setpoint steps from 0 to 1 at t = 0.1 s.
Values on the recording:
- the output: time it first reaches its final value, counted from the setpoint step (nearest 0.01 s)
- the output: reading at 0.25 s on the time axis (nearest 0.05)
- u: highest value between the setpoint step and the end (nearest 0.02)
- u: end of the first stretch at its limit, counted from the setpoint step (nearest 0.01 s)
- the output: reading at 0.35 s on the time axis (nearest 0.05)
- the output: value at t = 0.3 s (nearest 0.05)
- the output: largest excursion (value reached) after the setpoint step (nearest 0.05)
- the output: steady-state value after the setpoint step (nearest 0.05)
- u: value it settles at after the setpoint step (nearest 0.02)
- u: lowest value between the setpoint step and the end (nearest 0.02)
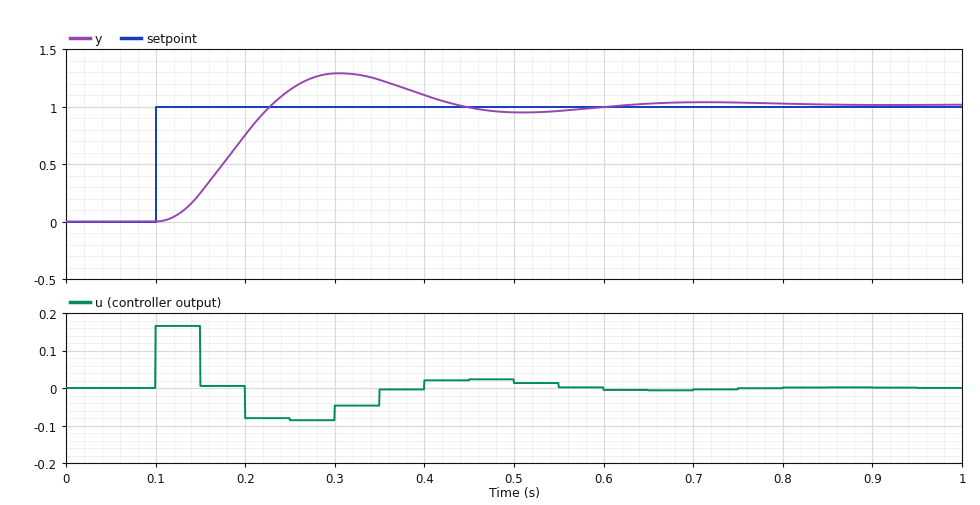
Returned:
0.13 s
1.15
0.16
0.05 s
1.25
1.30
1.30
1.00
0.00
-0.08
